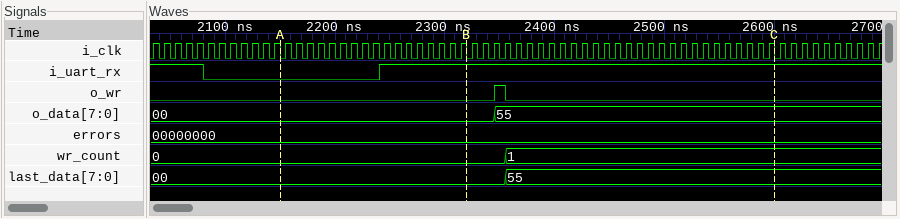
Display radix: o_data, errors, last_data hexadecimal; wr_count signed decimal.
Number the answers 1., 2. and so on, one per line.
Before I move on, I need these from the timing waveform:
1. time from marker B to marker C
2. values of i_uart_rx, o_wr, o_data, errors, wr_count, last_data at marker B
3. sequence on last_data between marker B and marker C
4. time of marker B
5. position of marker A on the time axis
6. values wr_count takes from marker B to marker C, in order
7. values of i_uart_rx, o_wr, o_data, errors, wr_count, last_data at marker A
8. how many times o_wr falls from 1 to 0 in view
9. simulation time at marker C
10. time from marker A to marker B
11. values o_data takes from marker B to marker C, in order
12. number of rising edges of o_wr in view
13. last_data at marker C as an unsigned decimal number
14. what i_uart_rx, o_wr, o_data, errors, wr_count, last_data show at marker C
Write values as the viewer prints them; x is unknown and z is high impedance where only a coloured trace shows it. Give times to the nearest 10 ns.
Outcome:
1. 280 ns
2. i_uart_rx=1, o_wr=0, o_data=00, errors=00000000, wr_count=0, last_data=00
3. 00, 55
4. 2320 ns
5. 2150 ns
6. 0, 1
7. i_uart_rx=0, o_wr=0, o_data=00, errors=00000000, wr_count=0, last_data=00
8. 1
9. 2600 ns
10. 170 ns
11. 00, 55
12. 1
13. 85
14. i_uart_rx=1, o_wr=0, o_data=55, errors=00000000, wr_count=1, last_data=55
